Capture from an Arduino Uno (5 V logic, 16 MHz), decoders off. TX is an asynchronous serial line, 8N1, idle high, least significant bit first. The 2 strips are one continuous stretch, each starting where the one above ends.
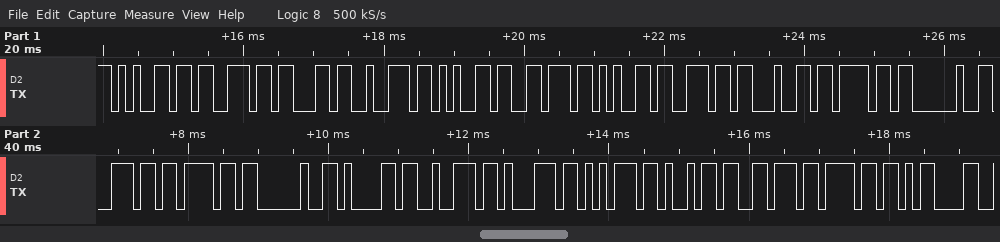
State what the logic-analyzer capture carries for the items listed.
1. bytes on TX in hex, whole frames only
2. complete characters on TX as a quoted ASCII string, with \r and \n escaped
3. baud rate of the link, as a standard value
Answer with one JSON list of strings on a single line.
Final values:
["65 73 63 72 65 76 65 6E 64 6F 20 6E 6F 20 61 72 71 75 69 76 6F 0D", "\"escrevendo no arquivo\\r\"", "9600 baud"]
